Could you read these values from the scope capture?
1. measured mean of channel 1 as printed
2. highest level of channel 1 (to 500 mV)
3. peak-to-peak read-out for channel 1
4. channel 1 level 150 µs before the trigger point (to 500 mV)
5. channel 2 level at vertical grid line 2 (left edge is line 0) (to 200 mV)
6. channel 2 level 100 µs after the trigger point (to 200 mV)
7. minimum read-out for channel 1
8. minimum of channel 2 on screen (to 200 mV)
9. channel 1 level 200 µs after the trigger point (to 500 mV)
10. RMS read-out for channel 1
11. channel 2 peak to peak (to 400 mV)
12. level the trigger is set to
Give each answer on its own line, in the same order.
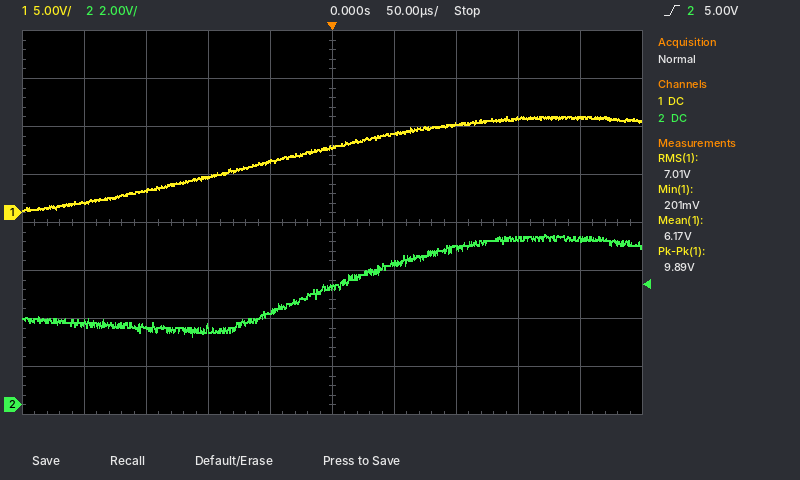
6.17 V
10.0 V
9.89 V
2.5 V
3.2 V
6.6 V
201 mV
2.8 V
10.0 V
7.01 V
4.4 V
5.00 V
